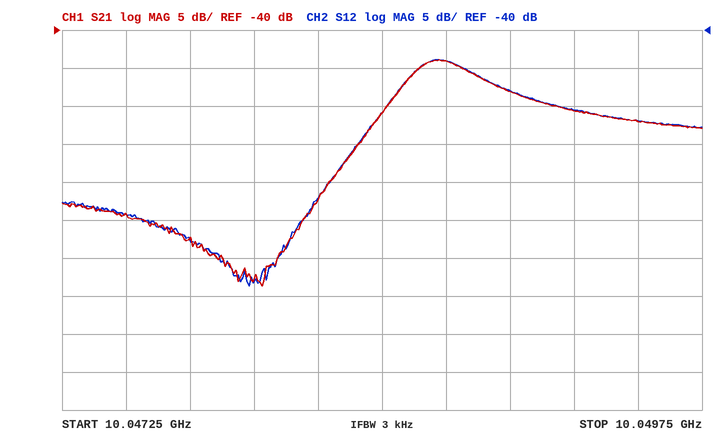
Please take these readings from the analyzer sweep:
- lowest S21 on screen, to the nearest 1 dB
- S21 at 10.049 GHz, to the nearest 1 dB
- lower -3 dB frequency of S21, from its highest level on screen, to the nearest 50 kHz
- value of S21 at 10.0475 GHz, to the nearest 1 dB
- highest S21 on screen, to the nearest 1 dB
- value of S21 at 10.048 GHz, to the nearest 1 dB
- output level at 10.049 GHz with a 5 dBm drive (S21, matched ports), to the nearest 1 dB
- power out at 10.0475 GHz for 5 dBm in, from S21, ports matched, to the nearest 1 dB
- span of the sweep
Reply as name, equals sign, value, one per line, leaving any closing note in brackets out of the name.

lowest S21 on screen, to the nearest 1 dB = -74 dB
S21 at 10.049 GHz, to the nearest 1 dB = -48 dB
lower -3 dB frequency of S21, from its highest level on screen, to the nearest 50 kHz = 10.04860 GHz
value of S21 at 10.0475 GHz, to the nearest 1 dB = -64 dB
highest S21 on screen, to the nearest 1 dB = -44 dB
value of S21 at 10.048 GHz, to the nearest 1 dB = -73 dB
output level at 10.049 GHz with a 5 dBm drive (S21, matched ports), to the nearest 1 dB = -43 dBm
power out at 10.0475 GHz for 5 dBm in, from S21, ports matched, to the nearest 1 dB = -59 dBm
span of the sweep = 2.5 MHz
